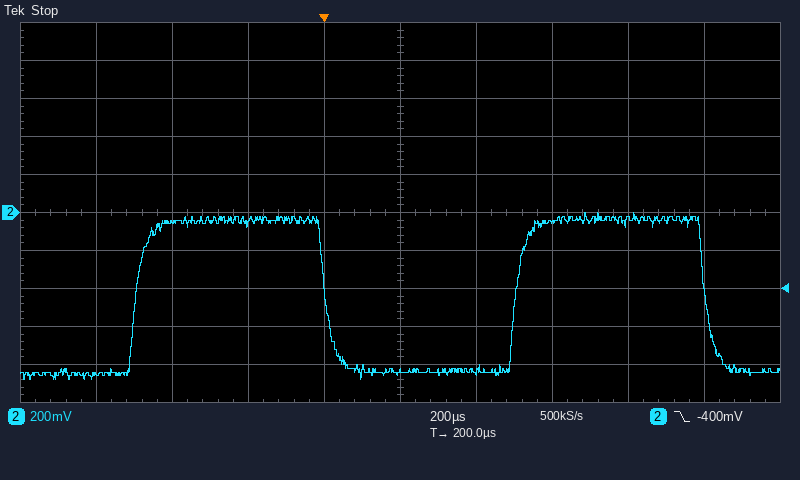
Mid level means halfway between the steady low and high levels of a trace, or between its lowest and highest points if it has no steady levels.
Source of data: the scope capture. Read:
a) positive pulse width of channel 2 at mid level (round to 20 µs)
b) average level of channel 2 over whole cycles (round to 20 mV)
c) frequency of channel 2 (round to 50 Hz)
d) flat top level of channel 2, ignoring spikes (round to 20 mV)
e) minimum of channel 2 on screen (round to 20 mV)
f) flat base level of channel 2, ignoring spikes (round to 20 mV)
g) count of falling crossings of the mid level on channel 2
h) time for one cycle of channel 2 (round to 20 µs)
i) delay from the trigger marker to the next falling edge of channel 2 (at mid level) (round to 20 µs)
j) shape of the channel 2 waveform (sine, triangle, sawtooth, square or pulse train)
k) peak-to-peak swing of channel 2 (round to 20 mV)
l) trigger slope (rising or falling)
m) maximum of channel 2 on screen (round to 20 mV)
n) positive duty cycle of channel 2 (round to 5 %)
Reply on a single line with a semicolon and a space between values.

500 µs; -440 mV; 1.00 kHz; -40 mV; -880 mV; -840 mV; 2; 1.00 ms; 1.00 ms; square; 880 mV; falling; 0 mV; 50 %
